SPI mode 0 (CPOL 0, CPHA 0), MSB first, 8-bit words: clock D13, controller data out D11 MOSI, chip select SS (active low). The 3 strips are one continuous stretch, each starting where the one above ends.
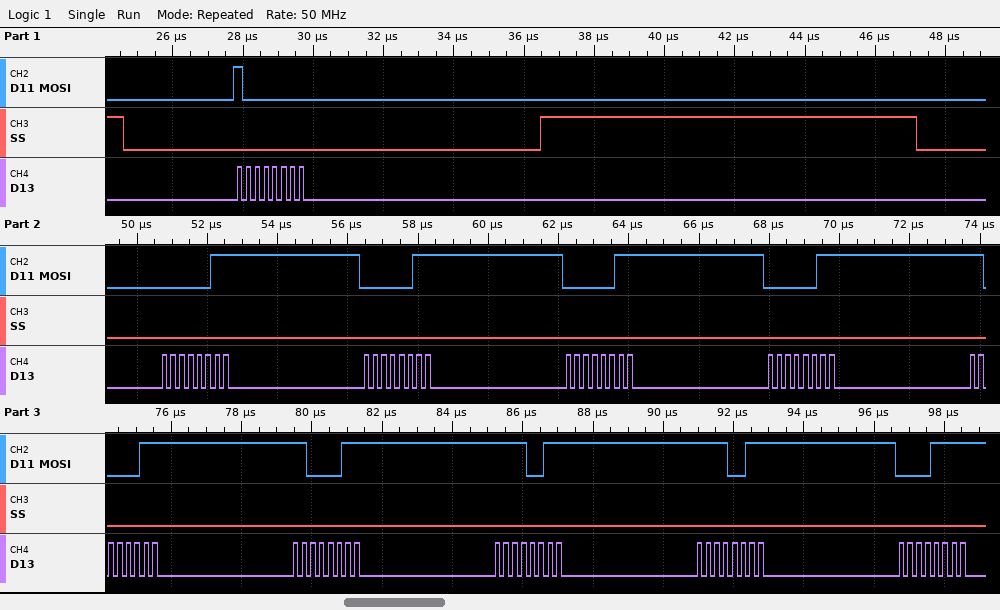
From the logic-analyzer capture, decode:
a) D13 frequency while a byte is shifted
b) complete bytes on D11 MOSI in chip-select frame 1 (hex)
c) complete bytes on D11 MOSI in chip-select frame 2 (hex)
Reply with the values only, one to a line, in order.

4 MHz
80
03 03 03 03 C3 C3 F3 F3 0F
